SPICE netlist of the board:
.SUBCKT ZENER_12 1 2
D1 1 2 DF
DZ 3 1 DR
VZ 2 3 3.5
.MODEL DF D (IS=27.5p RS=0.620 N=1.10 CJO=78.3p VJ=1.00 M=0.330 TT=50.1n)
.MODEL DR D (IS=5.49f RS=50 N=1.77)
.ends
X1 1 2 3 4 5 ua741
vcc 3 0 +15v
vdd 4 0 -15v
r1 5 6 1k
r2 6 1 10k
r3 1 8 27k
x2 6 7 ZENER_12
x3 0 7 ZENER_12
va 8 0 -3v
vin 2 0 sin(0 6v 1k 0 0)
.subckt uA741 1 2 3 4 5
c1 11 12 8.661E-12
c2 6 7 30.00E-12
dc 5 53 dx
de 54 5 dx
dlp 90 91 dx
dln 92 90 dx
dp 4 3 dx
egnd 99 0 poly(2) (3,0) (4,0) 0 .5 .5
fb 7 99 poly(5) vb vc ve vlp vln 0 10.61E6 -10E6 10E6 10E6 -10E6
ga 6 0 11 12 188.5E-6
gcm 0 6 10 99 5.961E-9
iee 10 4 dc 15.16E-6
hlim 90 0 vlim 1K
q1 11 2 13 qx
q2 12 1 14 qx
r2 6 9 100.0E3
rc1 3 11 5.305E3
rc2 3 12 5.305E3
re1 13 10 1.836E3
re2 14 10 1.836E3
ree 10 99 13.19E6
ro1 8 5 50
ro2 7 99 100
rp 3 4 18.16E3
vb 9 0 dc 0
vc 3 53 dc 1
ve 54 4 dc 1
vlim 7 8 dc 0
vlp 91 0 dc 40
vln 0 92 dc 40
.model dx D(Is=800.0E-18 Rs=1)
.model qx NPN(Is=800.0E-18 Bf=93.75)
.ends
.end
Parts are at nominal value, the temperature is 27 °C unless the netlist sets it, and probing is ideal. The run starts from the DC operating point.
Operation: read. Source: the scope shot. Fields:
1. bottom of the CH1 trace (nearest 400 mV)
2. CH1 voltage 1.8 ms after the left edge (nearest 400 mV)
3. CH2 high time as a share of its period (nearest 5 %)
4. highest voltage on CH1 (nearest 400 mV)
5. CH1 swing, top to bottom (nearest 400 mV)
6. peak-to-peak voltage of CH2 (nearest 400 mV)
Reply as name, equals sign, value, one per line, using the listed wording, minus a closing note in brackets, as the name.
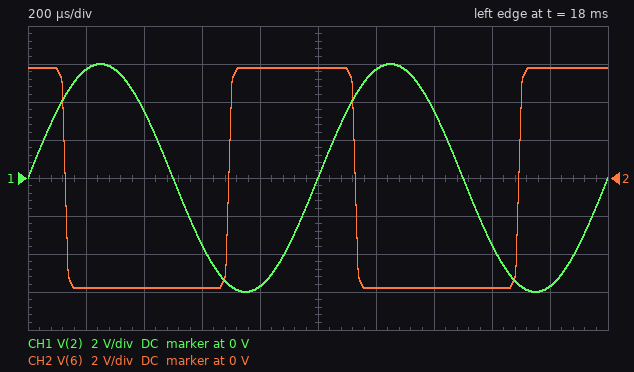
bottom of the CH1 trace = -6.0 V
CH1 voltage 1.8 ms after the left edge = -5.6 V
CH2 high time as a share of its period = 45 %
highest voltage on CH1 = 6.0 V
CH1 swing, top to bottom = 12.0 V
peak-to-peak voltage of CH2 = 11.6 V
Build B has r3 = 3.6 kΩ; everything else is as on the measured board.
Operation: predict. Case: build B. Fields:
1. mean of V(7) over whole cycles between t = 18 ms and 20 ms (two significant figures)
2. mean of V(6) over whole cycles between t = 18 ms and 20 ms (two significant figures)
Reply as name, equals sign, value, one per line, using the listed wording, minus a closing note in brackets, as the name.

mean of V(7) over whole cycles between t = 18 ms and 20 ms = 1.6 V
mean of V(6) over whole cycles between t = 18 ms and 20 ms = -1.5 V
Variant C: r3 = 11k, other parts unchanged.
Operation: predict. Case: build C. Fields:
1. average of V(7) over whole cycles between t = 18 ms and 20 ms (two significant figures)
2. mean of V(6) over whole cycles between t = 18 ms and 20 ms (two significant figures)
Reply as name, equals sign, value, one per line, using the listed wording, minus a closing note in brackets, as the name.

average of V(7) over whole cycles between t = 18 ms and 20 ms = 1.8 V
mean of V(6) over whole cycles between t = 18 ms and 20 ms = -1.1 V
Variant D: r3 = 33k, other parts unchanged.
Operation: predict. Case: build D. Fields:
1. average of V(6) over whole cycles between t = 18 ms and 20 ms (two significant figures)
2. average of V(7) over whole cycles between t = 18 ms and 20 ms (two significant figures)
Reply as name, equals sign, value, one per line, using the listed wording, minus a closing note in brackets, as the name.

average of V(6) over whole cycles between t = 18 ms and 20 ms = -680 mV
average of V(7) over whole cycles between t = 18 ms and 20 ms = 2.0 V
